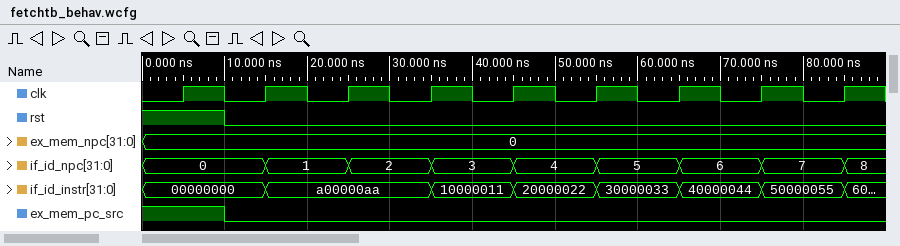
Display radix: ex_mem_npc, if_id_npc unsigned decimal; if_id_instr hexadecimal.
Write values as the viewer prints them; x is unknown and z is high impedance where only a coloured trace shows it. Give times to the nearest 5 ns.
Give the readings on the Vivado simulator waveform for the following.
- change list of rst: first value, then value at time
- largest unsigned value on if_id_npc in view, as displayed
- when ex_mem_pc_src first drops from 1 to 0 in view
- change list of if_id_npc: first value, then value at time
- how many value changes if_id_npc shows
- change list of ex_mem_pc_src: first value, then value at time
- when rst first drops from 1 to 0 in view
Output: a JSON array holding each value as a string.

["1, 0 at 10 ns", "8", "10 ns", "0, 1 at 15 ns, 2 at 25 ns, 3 at 35 ns, 4 at 45 ns, 5 at 55 ns, 6 at 65 ns, 7 at 75 ns, 8 at 85 ns", "8", "1, 0 at 10 ns", "10 ns"]
